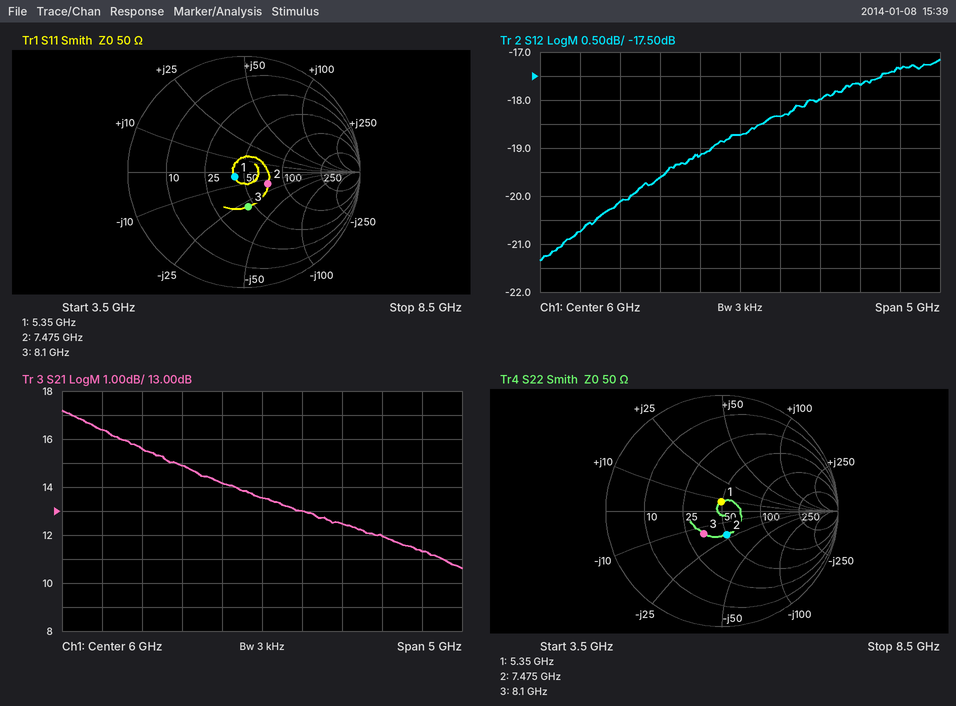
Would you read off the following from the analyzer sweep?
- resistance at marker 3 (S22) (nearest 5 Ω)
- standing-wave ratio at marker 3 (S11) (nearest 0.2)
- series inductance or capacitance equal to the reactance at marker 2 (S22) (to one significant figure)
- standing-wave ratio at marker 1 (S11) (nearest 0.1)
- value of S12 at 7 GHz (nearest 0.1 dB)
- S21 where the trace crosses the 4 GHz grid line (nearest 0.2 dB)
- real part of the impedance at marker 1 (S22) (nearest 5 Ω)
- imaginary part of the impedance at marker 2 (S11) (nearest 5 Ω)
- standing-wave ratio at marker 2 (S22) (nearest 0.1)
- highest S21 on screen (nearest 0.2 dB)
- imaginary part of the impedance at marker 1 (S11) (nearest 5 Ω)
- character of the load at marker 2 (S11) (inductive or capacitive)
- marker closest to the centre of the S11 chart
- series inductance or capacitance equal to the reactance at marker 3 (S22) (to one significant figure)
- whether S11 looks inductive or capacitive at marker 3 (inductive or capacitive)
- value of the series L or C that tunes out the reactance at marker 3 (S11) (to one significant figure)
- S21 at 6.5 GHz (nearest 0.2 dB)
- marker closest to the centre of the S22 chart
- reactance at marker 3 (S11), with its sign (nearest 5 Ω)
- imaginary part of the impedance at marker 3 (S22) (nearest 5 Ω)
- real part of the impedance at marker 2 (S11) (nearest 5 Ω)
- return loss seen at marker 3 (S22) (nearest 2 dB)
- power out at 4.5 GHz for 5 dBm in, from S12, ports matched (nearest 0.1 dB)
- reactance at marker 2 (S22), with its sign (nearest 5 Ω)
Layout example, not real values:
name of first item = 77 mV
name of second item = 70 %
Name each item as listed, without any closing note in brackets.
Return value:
resistance at marker 3 (S22) = 35 Ω
standing-wave ratio at marker 3 (S11) = 1.8
series inductance or capacitance equal to the reactance at marker 2 (S22) = 1 pF
standing-wave ratio at marker 1 (S11) = 1.2
value of S12 at 7 GHz = -18.0 dB
S21 where the trace crosses the 4 GHz grid line = 16.4 dB
real part of the impedance at marker 1 (S22) = 50 Ω
imaginary part of the impedance at marker 2 (S11) = -15 Ω
standing-wave ratio at marker 2 (S22) = 1.5
highest S21 on screen = 17.2 dB
imaginary part of the impedance at marker 1 (S11) = -5 Ω
character of the load at marker 2 (S11) = capacitive
marker closest to the centre of the S11 chart = marker 1
series inductance or capacitance equal to the reactance at marker 3 (S22) = 1 pF
whether S11 looks inductive or capacitive at marker 3 = capacitive
value of the series L or C that tunes out the reactance at marker 3 (S11) = 600 pH
S21 at 6.5 GHz = 13.0 dB
marker closest to the centre of the S22 chart = marker 1
reactance at marker 3 (S11), with its sign = -30 Ω
imaginary part of the impedance at marker 3 (S22) = -15 Ω
real part of the impedance at marker 2 (S11) = 75 Ω
return loss seen at marker 3 (S22) = 12 dB
power out at 4.5 GHz for 5 dBm in, from S12, ports matched = -15.1 dBm
reactance at marker 2 (S22), with its sign = -20 Ω
